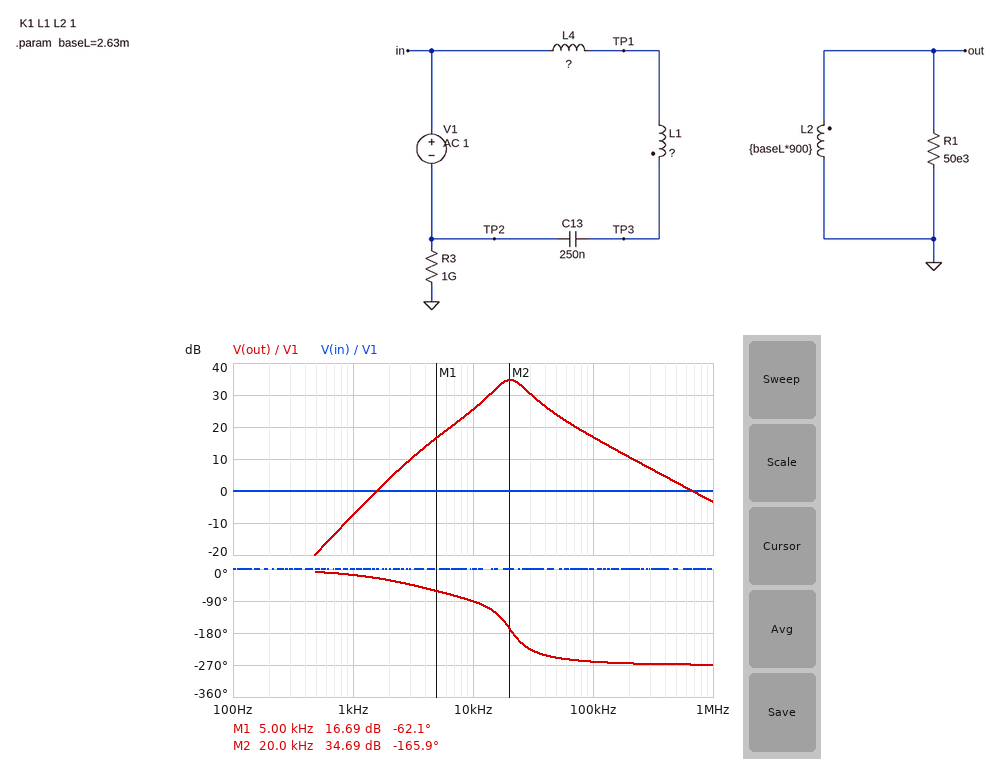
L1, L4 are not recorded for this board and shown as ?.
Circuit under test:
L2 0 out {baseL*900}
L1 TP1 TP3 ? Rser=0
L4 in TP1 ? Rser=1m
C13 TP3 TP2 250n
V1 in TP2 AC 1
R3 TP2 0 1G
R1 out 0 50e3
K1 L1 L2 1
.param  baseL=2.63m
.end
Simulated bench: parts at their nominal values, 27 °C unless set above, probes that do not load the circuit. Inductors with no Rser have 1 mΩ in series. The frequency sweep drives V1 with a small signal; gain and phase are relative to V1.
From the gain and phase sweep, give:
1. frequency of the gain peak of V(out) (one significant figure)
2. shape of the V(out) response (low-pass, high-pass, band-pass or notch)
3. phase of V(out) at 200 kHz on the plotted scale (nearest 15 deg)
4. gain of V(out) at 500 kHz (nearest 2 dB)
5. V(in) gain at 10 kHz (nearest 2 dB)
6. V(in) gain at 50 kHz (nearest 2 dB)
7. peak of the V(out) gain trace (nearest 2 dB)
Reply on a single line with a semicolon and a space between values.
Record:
20 kHz; band-pass; -270 deg; 2 dB; 0 dB; 0 dB; 34 dB
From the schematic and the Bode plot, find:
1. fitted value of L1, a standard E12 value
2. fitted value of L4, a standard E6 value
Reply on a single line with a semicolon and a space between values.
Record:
820 µH; 220 µH
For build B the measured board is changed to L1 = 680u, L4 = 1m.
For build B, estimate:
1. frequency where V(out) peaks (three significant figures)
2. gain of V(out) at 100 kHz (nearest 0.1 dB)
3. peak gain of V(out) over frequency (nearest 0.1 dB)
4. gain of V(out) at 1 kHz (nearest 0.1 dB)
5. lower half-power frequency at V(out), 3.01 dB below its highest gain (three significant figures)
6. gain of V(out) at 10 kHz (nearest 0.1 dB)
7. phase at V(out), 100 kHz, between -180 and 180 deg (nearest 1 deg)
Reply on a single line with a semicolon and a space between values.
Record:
9.71 kHz; 2.7 dB; 35.9 dB; -8.3 dB; 8.76 kHz; 35.6 dB; 93 deg
